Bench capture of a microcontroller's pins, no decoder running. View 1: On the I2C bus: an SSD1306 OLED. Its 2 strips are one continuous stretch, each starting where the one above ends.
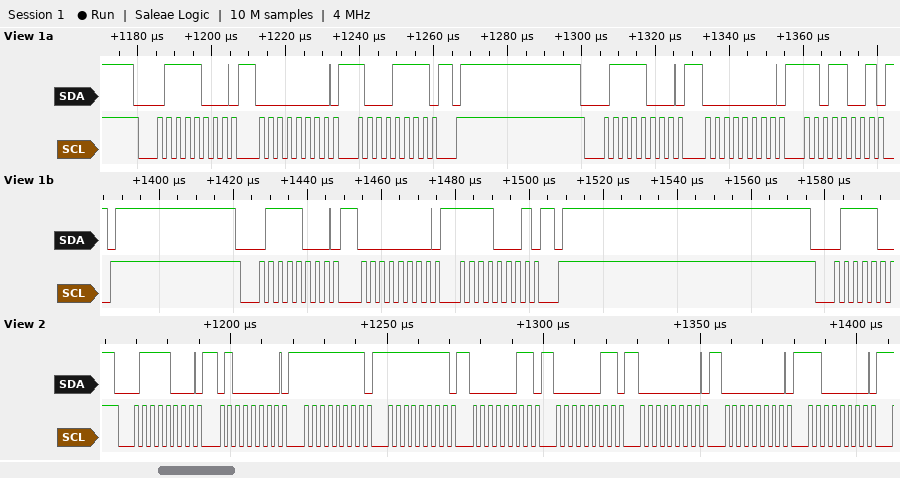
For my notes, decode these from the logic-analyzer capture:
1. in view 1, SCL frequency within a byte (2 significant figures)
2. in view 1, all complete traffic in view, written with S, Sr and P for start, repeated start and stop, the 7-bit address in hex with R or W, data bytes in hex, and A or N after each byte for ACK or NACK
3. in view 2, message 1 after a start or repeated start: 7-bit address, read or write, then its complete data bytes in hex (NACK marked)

400 kHz
S 3CW A 00 A 8F A P S 3CW A 00 A D9 A P S 3CW A 00 A F1 A P
0x3C write: 40 FF FF 03 03 00 00 C0
